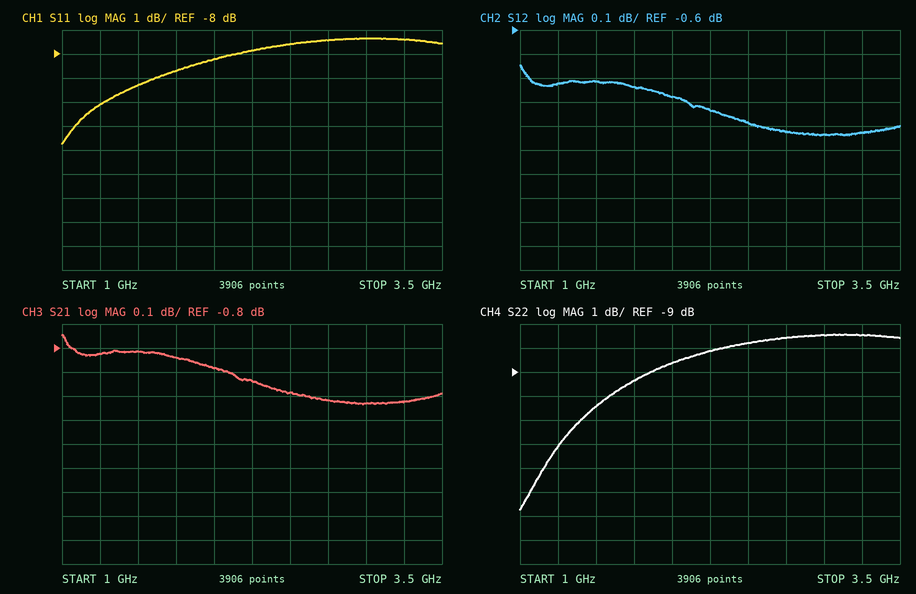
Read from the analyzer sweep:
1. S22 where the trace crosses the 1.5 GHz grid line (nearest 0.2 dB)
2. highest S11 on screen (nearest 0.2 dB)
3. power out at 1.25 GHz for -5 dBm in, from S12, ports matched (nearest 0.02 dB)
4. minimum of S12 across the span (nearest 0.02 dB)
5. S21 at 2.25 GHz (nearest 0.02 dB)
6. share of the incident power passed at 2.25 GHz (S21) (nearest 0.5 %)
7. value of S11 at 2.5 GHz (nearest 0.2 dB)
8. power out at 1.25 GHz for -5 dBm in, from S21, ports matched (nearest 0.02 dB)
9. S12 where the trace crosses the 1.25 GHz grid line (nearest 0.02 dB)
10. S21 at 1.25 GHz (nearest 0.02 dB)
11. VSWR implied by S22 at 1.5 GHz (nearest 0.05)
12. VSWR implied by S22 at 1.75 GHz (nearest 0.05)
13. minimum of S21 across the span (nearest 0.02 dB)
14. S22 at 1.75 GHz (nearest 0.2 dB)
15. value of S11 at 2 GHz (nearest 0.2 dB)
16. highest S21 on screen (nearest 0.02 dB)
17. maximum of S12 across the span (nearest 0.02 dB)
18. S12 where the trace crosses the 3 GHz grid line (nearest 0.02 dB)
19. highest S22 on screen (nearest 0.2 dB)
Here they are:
-10.4 dB
-7.4 dB
-5.82 dBm
-1.04 dB
-0.94 dB
80.5 %
-7.6 dB
-5.82 dBm
-0.82 dB
-0.82 dB
1.85
2.05
-1.04 dB
-9.4 dB
-8.2 dB
-0.74 dB
-0.74 dB
-1.04 dB
-7.4 dB
